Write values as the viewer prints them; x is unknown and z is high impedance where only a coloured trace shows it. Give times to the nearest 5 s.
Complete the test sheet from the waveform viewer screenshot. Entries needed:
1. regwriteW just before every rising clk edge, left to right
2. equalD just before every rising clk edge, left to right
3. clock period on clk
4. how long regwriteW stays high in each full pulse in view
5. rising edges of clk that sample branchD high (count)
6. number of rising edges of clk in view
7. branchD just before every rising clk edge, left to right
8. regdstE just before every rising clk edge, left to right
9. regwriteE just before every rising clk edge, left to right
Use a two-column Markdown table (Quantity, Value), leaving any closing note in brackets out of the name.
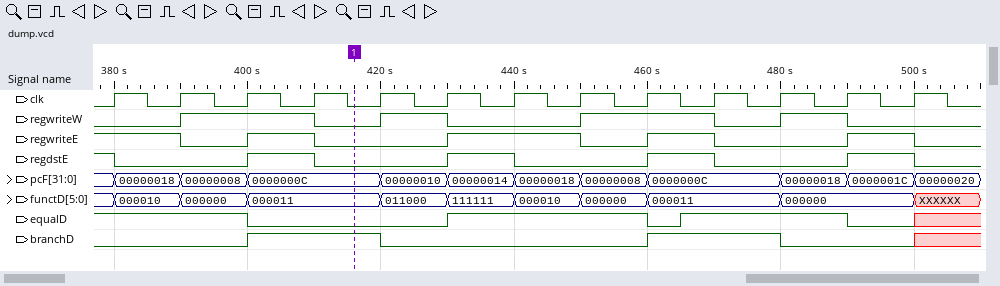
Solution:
| Quantity | Value |
|---|---|
| regwriteW just before every rising clk edge, left to right | 0 0 1 1 0 1 0 0 1 1 0 1 0 |
| equalD just before every rising clk edge, left to right | 1 1 1 0 0 0 1 1 1 1 1 1 0 |
| clock period on clk | 10 s |
| how long regwriteW stays high in each full pulse in view | 20 s, 10 s, 20 s, 10 s |
| rising edges of clk that sample branchD high | 4 |
| number of rising edges of clk in view | 13 |
| branchD just before every rising clk edge, left to right | 0 0 0 1 1 0 0 0 0 1 1 0 0 |
| regdstE just before every rising clk edge, left to right | 1 0 0 1 0 0 1 0 0 1 0 0 1 |
| regwriteE just before every rising clk edge, left to right | 1 1 0 1 0 0 1 1 0 1 0 0 1 |
